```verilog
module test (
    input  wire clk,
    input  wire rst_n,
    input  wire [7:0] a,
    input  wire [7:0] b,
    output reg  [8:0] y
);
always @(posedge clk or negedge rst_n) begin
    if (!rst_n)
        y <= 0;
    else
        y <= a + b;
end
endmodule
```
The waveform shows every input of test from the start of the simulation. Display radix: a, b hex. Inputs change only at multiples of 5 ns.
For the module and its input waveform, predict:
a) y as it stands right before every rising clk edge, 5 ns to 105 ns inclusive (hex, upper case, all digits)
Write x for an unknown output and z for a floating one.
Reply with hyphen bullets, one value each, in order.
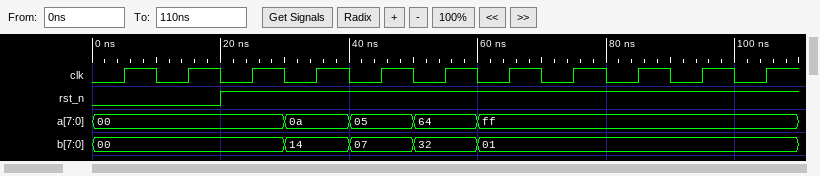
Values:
- 000, 000, 000, 000, 01E, 00C, 096, 100, 100, 100, 100
